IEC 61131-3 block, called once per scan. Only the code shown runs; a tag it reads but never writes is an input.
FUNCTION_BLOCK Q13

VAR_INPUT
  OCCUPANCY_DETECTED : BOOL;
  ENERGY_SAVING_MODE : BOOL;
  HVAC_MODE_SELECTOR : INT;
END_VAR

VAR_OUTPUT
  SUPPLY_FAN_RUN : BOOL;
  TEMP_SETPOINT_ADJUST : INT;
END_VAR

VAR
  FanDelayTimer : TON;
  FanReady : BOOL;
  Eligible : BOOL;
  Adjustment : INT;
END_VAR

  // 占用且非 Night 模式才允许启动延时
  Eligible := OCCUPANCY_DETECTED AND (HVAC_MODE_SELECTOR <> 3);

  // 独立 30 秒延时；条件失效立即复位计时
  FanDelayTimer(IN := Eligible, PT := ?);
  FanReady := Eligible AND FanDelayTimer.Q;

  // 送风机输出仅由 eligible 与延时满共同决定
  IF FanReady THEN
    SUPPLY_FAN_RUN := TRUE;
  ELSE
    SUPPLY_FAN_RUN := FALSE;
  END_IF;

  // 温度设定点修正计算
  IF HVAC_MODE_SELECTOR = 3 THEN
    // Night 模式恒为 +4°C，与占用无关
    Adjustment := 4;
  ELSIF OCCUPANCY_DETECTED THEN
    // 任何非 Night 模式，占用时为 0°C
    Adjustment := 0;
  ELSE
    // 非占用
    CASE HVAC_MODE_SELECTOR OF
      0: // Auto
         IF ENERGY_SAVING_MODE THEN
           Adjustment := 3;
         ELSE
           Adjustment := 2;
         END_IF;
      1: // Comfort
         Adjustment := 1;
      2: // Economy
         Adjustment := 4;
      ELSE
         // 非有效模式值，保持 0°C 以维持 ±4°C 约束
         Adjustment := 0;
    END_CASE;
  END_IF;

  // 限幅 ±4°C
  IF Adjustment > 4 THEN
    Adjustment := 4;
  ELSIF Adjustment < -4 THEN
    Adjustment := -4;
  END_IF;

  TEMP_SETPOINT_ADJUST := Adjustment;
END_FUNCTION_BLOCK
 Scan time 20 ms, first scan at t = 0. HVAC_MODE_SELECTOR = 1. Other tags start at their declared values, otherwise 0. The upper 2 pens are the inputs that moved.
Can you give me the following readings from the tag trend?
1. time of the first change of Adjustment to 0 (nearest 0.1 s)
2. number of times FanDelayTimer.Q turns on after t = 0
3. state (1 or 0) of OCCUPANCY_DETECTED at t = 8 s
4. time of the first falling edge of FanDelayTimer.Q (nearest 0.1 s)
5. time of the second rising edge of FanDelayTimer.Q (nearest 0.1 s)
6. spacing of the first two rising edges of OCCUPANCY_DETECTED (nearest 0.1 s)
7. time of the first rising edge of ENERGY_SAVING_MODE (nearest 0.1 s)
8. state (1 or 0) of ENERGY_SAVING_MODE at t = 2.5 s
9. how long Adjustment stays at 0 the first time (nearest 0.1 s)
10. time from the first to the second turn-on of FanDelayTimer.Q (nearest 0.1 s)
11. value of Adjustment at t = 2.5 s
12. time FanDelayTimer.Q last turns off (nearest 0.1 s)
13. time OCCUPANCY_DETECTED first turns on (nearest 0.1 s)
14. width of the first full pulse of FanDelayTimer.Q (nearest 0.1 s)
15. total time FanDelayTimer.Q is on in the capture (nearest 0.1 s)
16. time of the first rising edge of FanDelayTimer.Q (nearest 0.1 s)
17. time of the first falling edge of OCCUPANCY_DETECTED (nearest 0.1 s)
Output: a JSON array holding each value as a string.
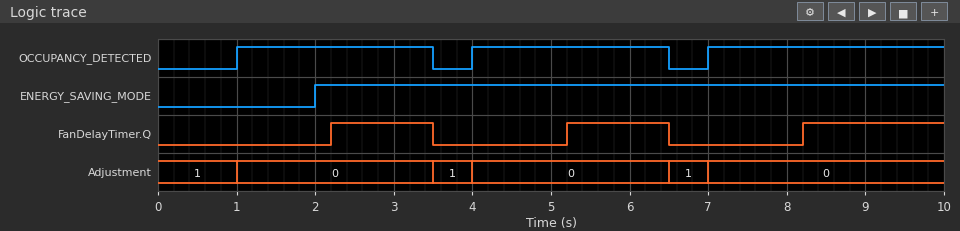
["1.0 s", "3", "1", "3.5 s", "5.2 s", "3.0 s", "2.0 s", "1", "2.5 s", "3.0 s", "0", "6.5 s", "1.0 s", "1.3 s", "4.4 s", "2.2 s", "3.5 s"]
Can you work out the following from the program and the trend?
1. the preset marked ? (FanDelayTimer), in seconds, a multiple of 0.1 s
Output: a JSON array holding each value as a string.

["1.2 s"]
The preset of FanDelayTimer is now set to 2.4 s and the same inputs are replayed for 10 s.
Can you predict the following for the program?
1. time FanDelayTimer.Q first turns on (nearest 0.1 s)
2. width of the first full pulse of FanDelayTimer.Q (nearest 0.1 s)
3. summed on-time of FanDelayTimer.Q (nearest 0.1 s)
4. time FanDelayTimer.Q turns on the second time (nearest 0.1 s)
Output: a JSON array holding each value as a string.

["3.4 s", "0.1 s", "0.8 s", "6.4 s"]
